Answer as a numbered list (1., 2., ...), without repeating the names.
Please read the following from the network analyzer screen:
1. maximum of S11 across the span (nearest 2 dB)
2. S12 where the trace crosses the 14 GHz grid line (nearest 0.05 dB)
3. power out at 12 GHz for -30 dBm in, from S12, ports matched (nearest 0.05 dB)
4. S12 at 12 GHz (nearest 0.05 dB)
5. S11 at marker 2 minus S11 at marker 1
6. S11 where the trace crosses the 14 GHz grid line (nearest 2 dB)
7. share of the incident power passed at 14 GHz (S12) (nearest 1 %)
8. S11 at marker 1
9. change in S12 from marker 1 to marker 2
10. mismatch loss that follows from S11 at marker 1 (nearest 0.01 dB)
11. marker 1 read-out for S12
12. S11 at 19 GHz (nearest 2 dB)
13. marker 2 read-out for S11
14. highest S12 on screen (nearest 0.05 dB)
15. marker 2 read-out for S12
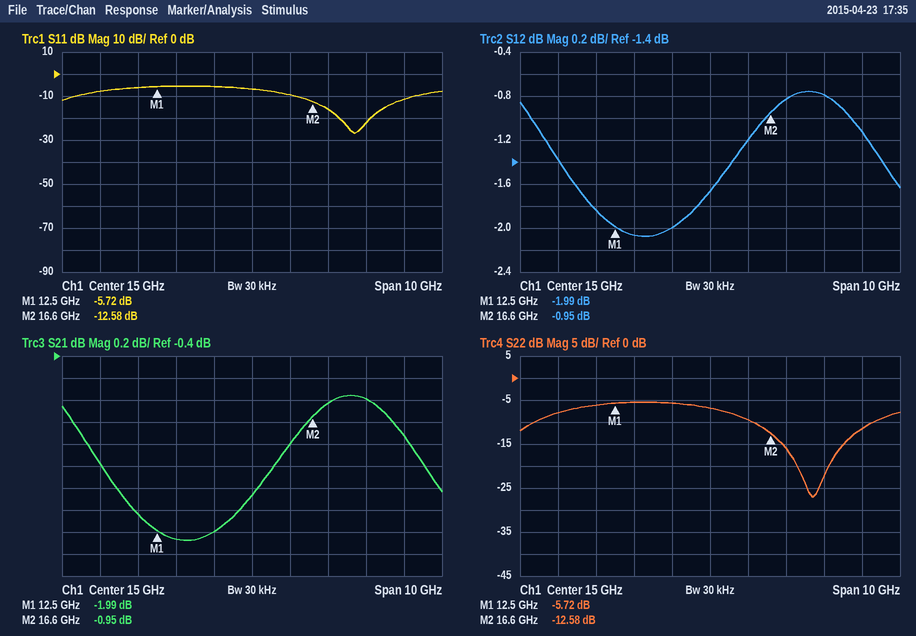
1. -6 dB
2. -2.00 dB
3. -31.85 dBm
4. -1.85 dB
5. -6.86 dB
6. -6 dB
7. 63 %
8. -5.72 dB
9. 1.04 dB
10. 1.35 dB
11. -1.99 dB
12. -12 dB
13. -12.58 dB
14. -0.75 dB
15. -0.95 dB
